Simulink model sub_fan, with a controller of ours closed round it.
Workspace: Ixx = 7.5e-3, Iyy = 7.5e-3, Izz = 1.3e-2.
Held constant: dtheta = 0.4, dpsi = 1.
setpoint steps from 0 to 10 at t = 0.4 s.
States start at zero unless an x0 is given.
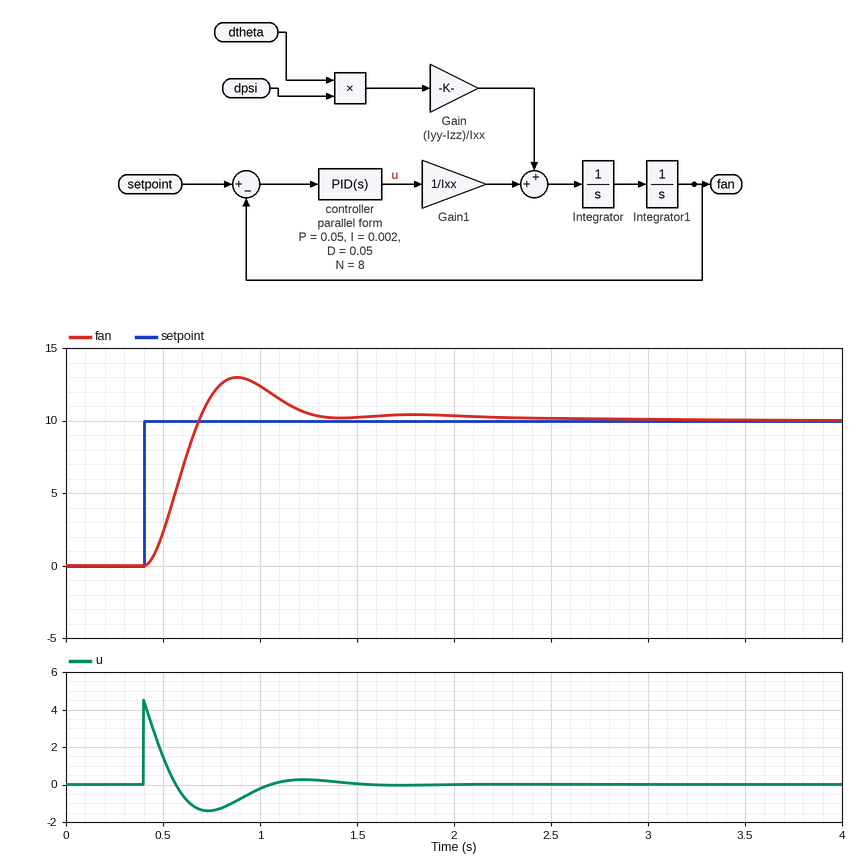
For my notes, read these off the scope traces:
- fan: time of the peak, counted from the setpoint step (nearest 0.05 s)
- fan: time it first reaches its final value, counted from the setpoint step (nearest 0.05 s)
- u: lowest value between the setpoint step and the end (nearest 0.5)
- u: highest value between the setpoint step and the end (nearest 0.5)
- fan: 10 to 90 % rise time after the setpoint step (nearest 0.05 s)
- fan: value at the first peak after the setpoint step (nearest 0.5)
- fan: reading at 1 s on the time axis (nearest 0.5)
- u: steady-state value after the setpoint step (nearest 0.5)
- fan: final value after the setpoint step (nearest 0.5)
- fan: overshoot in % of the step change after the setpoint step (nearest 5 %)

0.50 s
0.30 s
-1.5
4.5
0.20 s
13.0
12.5
0.0
10.0
30 %
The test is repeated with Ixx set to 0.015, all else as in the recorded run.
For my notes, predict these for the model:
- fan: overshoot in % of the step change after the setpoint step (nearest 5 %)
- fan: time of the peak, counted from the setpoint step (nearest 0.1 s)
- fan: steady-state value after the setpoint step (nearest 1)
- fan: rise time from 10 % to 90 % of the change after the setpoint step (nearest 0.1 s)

25 %
0.8 s
10
0.3 s
